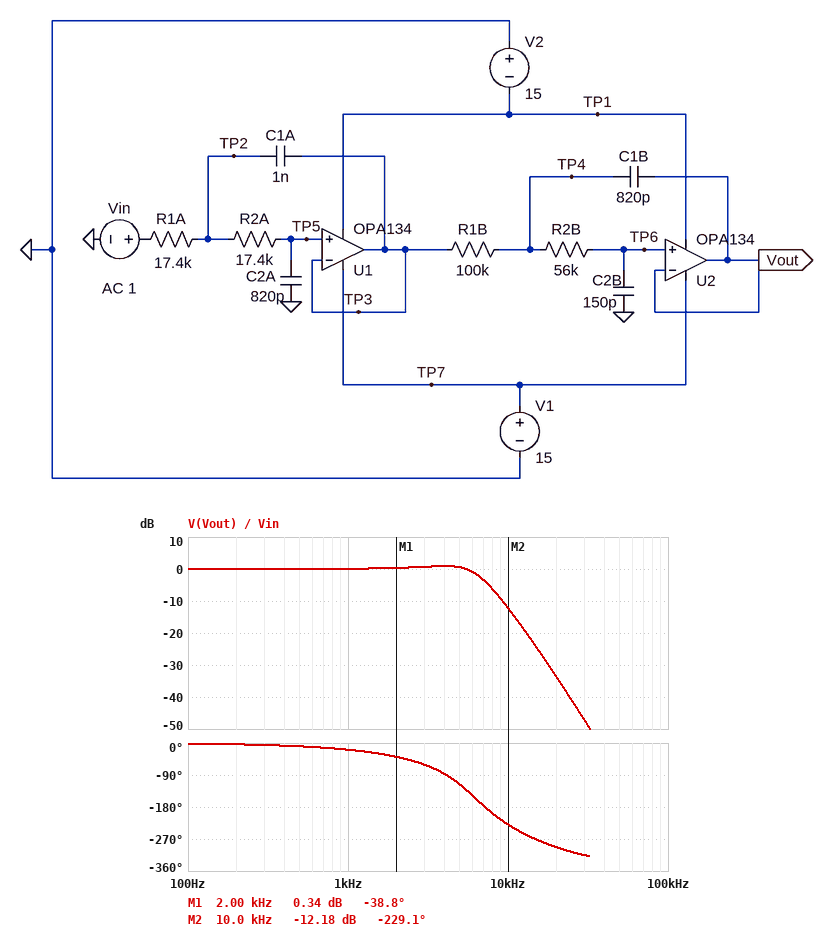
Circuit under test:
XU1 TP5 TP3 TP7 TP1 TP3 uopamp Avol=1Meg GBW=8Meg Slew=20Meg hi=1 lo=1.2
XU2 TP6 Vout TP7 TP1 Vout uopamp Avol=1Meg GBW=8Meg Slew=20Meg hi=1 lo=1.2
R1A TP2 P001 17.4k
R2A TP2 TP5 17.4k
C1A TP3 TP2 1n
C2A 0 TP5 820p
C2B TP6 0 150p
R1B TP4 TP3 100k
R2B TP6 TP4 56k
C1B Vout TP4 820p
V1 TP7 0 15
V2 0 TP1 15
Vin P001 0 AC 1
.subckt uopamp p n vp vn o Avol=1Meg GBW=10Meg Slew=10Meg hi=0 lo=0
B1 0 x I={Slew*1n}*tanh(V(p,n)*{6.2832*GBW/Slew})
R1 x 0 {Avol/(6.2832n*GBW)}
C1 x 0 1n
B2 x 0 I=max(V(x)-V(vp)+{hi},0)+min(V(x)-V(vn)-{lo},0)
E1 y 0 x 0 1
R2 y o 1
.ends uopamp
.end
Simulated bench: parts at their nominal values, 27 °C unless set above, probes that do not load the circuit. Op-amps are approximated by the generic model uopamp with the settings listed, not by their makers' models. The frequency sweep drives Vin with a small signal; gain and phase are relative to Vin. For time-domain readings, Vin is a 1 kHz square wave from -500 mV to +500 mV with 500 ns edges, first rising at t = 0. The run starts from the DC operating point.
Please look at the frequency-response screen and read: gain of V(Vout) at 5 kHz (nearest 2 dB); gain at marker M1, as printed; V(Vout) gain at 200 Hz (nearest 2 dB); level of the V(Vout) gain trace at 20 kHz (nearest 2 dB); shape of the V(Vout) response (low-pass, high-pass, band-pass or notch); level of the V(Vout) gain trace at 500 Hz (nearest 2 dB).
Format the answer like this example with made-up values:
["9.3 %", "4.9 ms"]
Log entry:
["0 dB", "0.34 dB", "0 dB", "-34 dB", "low-pass", "0 dB"]
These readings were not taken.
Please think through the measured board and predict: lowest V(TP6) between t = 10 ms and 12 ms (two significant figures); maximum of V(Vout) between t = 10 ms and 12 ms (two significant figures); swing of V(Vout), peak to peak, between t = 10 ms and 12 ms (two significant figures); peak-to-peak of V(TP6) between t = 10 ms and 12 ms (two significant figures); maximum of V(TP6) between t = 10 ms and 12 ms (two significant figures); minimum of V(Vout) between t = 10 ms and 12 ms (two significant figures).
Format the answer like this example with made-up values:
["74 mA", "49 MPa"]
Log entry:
["-660 mV", "660 mV", "1.3 V", "1.3 V", "660 mV", "-660 mV"]
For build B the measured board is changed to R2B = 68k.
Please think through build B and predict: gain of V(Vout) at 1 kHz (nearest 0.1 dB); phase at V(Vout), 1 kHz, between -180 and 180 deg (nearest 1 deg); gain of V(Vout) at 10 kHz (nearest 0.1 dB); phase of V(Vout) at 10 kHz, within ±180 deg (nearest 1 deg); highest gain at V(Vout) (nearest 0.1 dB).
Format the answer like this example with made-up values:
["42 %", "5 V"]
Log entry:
["0.1 dB", "-20 deg", "-14.0 dB", "125 deg", "1.2 dB"]
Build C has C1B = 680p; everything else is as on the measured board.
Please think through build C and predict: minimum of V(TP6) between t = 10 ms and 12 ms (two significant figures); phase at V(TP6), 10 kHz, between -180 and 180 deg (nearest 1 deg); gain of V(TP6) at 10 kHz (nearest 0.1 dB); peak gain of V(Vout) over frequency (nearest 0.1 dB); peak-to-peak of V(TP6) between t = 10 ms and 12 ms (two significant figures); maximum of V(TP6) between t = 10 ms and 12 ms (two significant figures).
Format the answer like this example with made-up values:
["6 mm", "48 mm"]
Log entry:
["-620 mV", "140 deg", "-10.8 dB", "0.4 dB", "1.2 V", "620 mV"]
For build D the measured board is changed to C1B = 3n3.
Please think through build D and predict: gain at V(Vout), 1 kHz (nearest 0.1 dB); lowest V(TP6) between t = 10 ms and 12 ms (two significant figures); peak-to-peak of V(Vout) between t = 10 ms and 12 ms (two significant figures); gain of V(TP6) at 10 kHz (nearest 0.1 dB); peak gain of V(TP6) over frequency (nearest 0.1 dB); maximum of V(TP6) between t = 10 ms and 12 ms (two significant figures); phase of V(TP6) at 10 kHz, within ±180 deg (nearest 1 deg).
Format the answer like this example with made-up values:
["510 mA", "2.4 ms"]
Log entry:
["0.8 dB", "-1.0 V", "2.0 V", "-25.1 dB", "6.8 dB", "1.0 V", "99 deg"]
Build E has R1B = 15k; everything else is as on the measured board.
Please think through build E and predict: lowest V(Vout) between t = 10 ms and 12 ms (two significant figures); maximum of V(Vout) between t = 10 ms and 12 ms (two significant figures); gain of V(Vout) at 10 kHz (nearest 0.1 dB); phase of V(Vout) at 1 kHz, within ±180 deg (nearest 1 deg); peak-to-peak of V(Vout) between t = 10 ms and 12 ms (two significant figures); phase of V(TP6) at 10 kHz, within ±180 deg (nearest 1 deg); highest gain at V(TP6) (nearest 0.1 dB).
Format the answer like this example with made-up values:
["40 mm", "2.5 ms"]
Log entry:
["-500 mV", "500 mV", "-4.1 dB", "-14 deg", "1.0 V", "-138 deg", "0 dB"]
